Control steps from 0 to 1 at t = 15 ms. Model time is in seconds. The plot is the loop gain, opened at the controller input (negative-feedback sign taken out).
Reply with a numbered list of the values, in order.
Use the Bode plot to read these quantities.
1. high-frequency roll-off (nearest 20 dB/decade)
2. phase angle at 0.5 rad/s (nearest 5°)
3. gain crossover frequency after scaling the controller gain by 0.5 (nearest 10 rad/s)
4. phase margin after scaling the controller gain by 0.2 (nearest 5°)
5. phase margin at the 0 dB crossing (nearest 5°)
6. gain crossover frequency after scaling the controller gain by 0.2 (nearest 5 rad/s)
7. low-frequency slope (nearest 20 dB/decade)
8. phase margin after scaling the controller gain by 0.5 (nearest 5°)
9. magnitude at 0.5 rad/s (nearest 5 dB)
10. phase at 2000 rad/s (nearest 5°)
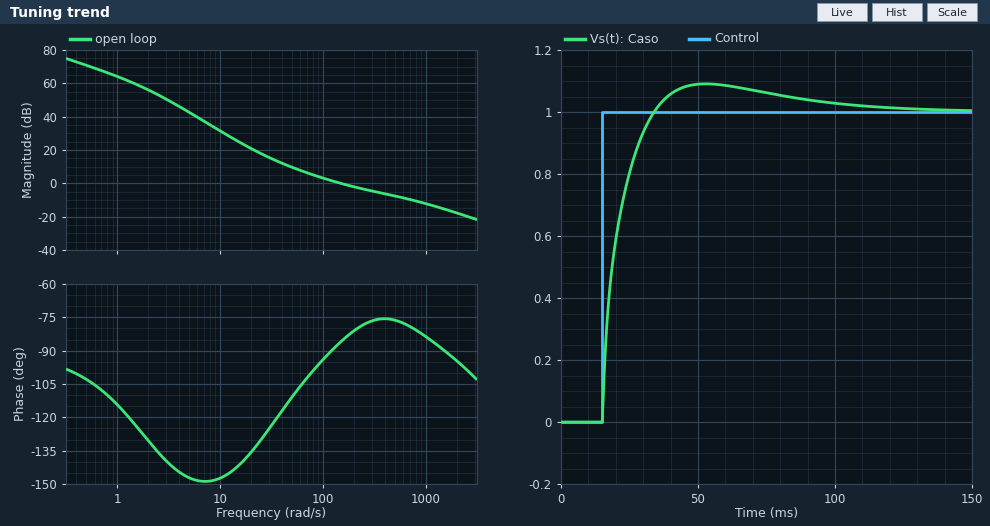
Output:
1. -20 dB/decade
2. -105°
3. 70 rad/s
4. 60°
5. 95°
6. 35 rad/s
7. -20 dB/decade
8. 80°
9. 70 dB
10. -95°
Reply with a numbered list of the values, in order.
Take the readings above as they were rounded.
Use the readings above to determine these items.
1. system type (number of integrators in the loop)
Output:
1. 1
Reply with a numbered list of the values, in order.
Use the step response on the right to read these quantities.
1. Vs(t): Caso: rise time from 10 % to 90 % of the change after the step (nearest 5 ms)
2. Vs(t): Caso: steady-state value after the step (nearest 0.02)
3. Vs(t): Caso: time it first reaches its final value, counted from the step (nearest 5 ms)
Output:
1. 15 ms
2. 1.00
3. 20 ms
